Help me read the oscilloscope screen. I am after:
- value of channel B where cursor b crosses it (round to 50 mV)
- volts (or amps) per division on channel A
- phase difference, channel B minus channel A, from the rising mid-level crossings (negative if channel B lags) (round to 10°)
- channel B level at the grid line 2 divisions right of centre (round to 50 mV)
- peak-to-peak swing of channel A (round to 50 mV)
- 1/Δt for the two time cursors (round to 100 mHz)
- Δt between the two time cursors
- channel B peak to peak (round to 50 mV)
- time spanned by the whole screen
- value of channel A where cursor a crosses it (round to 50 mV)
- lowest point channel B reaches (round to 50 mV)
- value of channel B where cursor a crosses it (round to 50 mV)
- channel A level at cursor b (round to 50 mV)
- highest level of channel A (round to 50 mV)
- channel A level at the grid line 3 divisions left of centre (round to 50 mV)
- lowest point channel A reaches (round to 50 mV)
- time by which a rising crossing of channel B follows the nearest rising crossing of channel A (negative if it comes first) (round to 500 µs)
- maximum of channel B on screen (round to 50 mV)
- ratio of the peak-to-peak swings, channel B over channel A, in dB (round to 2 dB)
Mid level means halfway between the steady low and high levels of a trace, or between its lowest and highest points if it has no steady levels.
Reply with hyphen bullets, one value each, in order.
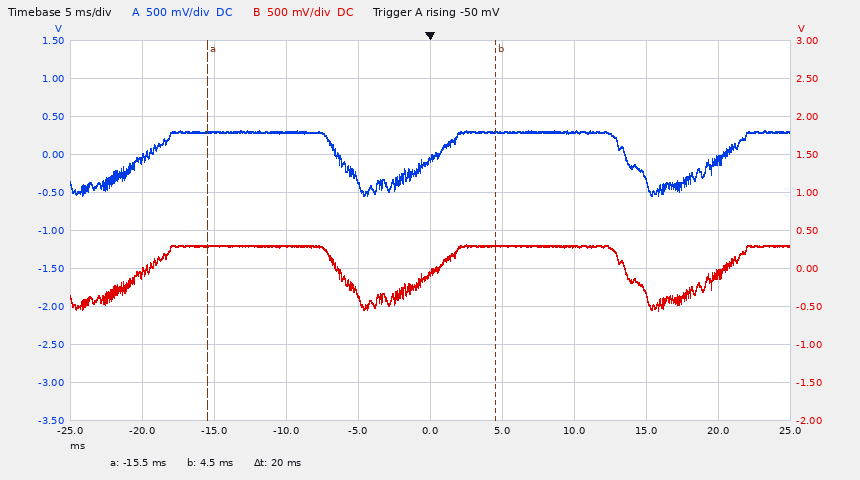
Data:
- 300 mV
- 500 mV
- 0°
- 300 mV
- 850 mV
- 50.0 Hz
- 20 ms
- 850 mV
- 50 ms
- 300 mV
- -550 mV
- 300 mV
- 300 mV
- 300 mV
- 300 mV
- -550 mV
- 0.0 ms
- 300 mV
- 0 dB
